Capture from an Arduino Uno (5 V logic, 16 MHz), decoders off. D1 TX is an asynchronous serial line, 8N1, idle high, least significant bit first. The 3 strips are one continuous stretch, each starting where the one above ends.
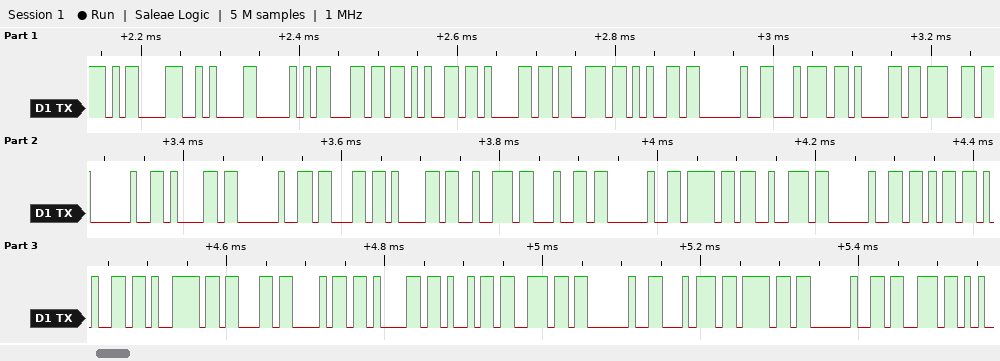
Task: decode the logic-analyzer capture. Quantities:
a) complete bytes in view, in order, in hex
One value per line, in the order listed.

0D 0A 50 6C 65 61 73 65 20 74 61 67 20 61 20 63 61 72 64 20 6F 72 20 6B 65 79 63 68 61 69 6E 20 74 6F 20 73
